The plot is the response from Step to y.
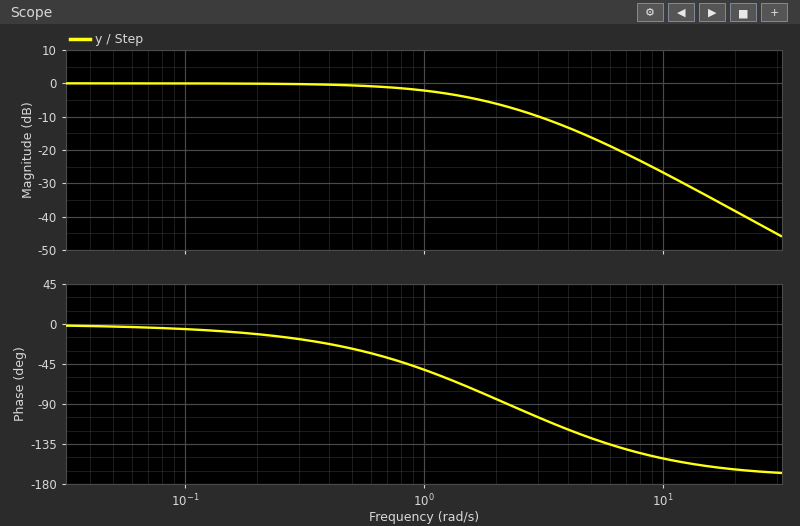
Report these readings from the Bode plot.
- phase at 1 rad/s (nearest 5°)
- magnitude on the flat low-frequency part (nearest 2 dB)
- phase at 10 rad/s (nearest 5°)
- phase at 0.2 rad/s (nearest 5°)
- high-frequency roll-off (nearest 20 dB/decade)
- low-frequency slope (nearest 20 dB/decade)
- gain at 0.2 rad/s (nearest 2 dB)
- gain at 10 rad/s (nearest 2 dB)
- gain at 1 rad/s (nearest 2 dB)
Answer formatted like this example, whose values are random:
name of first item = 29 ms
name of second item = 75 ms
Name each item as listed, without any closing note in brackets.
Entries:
phase at 1 rad/s = -50°
magnitude on the flat low-frequency part = 0 dB
phase at 10 rad/s = -150°
phase at 0.2 rad/s = -10°
high-frequency roll-off = -40 dB/decade
low-frequency slope = 0 dB/decade
gain at 0.2 rad/s = 0 dB
gain at 10 rad/s = -26 dB
gain at 1 rad/s = -2 dB
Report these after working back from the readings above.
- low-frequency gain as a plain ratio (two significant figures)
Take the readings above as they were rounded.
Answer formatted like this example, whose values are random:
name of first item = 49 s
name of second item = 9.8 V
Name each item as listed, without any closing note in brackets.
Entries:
low-frequency gain as a plain ratio = 1.0
